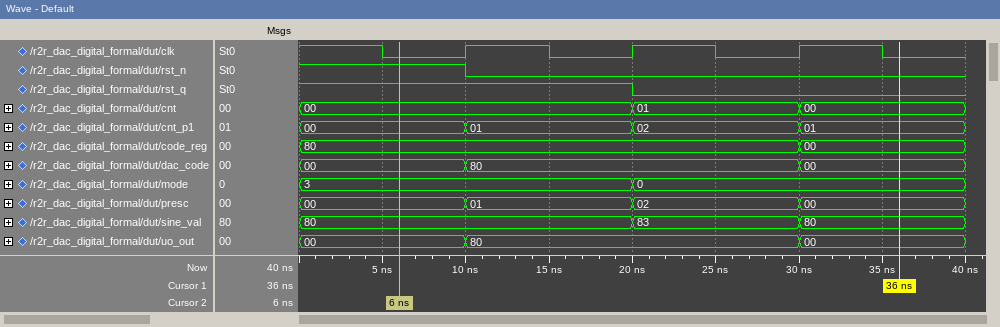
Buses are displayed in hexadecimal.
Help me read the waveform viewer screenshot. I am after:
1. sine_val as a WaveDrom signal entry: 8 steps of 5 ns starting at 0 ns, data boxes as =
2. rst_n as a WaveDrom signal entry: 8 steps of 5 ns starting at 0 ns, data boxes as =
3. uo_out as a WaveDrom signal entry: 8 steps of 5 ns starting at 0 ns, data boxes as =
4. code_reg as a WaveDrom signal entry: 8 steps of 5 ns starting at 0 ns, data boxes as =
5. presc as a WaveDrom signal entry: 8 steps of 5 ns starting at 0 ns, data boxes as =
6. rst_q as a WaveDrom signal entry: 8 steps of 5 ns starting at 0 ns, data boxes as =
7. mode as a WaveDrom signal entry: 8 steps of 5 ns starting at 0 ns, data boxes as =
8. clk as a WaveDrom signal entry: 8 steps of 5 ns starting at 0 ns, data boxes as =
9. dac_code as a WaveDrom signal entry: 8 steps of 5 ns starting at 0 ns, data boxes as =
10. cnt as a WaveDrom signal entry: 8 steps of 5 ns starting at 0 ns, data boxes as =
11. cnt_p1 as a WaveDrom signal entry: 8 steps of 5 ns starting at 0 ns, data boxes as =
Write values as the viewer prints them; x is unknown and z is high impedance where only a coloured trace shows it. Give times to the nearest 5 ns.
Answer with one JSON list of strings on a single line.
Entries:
["{name: 'sine_val', wave: '=...=.=.', data: '80 83 80'}", "{name: 'rst_n', wave: '1.0.....'}", "{name: 'uo_out', wave: '=.=...=.', data: '00 80 00'}", "{name: 'code_reg', wave: '=.....=.', data: '80 00'}", "{name: 'presc', wave: '=.=.=.=.', data: '00 01 02 00'}", "{name: 'rst_q', wave: '1...0...'}", "{name: 'mode', wave: '=...=...', data: '3 0'}", "{name: 'clk', wave: '10101010'}", "{name: 'dac_code', wave: '=.=...=.', data: '00 80 00'}", "{name: 'cnt', wave: '=...=.=.', data: '00 01 00'}", "{name: 'cnt_p1', wave: '=.=.=.=.', data: '00 01 02 01'}"]
